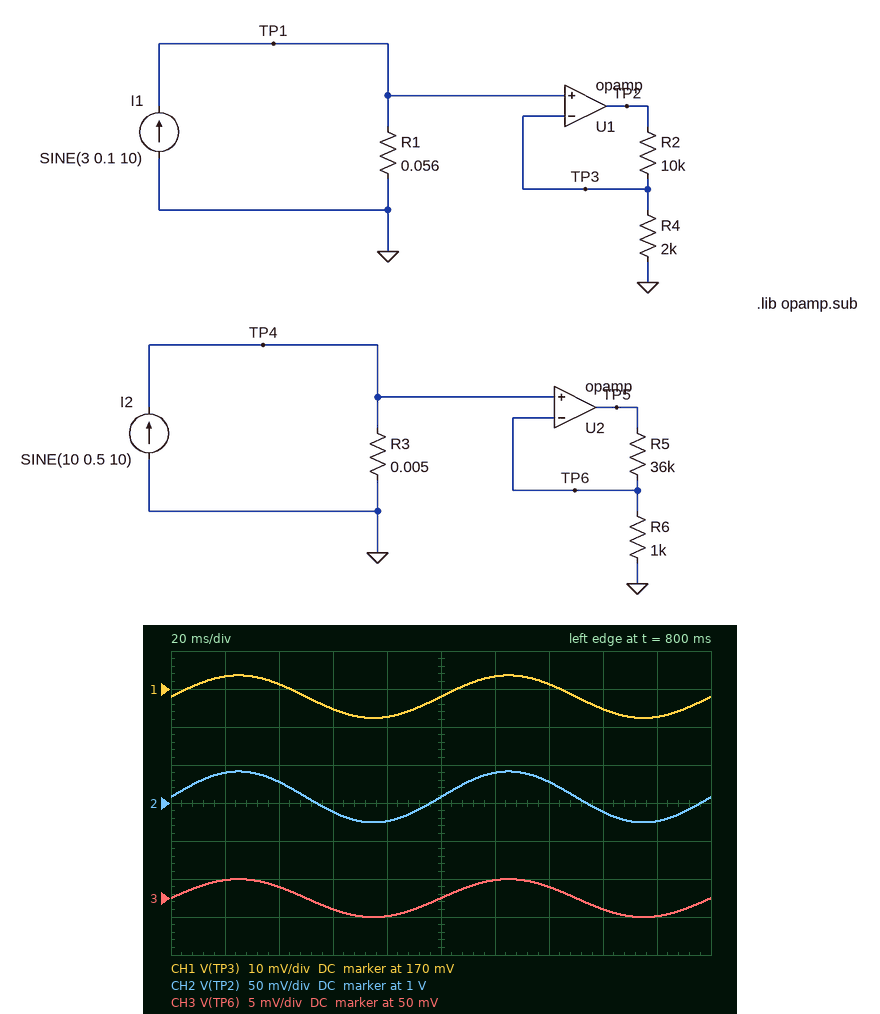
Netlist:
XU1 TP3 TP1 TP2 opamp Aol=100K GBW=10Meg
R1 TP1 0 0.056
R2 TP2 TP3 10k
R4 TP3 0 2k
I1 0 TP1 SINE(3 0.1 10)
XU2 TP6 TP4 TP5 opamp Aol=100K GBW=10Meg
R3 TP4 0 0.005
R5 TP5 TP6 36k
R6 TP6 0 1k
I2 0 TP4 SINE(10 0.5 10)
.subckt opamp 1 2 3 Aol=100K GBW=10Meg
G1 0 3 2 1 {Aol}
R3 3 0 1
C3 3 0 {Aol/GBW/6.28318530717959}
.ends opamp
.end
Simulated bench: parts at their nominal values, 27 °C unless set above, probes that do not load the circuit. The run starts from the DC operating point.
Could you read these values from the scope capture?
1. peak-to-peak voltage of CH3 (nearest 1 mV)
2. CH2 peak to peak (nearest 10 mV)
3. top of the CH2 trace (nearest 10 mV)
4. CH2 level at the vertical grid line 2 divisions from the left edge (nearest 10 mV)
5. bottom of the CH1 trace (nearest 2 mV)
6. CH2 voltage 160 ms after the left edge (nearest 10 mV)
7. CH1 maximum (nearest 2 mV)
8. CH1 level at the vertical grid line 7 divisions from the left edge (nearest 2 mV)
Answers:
5 mV
70 mV
1.04 V
1.03 V
162 mV
990 mV
174 mV
172 mV
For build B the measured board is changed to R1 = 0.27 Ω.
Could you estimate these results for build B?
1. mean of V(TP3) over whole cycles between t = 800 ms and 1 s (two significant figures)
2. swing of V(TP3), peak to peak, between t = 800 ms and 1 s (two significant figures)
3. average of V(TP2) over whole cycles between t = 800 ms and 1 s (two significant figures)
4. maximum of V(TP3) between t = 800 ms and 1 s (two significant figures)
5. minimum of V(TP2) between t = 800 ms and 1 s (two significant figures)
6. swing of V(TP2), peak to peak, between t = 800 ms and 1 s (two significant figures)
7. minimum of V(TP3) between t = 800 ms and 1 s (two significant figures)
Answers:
810 mV
54 mV
4.9 V
840 mV
4.7 V
320 mV
780 mV
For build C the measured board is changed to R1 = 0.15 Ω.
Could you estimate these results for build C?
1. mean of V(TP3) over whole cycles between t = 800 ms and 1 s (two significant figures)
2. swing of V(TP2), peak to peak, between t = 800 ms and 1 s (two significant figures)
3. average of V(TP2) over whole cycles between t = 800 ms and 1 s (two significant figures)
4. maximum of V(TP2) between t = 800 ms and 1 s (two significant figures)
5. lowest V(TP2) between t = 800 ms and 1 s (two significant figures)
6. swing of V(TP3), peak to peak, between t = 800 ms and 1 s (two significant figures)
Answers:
450 mV
180 mV
2.7 V
2.8 V
2.6 V
30 mV
